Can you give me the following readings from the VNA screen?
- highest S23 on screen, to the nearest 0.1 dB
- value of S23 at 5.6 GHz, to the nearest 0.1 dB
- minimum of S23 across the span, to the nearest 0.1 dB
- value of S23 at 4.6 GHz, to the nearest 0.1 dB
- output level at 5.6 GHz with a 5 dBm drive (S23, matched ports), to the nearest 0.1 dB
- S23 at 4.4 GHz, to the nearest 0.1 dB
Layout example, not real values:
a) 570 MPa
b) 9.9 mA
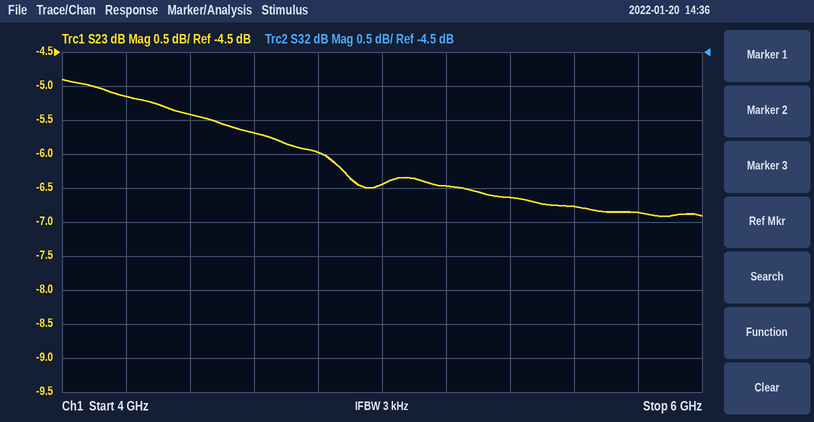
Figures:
a) -4.9 dB
b) -6.8 dB
c) -6.9 dB
d) -5.7 dB
e) -1.8 dBm
f) -5.4 dB
